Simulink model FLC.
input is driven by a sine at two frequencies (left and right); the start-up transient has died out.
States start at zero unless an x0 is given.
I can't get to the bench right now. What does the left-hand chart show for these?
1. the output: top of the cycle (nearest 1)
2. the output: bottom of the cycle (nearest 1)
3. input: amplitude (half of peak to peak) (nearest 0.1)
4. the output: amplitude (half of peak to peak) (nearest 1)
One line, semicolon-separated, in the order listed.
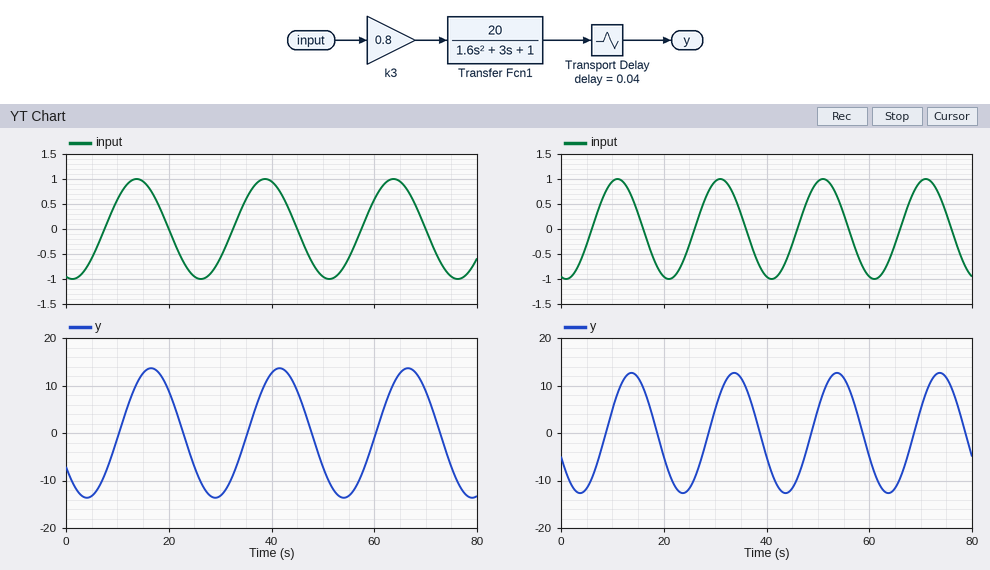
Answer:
14; -14; 1.0; 14
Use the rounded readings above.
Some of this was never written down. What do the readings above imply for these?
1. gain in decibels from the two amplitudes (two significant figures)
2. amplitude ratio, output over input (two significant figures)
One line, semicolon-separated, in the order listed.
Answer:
23 dB; 14
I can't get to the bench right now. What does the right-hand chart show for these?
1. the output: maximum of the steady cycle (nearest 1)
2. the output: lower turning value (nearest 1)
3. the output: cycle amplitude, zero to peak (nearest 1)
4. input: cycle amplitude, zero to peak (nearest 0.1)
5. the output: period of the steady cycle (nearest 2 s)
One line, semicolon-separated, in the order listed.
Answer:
13; -13; 13; 1.0; 20 s
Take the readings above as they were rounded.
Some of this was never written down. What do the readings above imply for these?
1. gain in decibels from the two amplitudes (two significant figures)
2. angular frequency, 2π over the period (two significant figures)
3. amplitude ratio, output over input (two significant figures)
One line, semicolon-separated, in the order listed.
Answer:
22 dB; 0.31 rad/s; 13
